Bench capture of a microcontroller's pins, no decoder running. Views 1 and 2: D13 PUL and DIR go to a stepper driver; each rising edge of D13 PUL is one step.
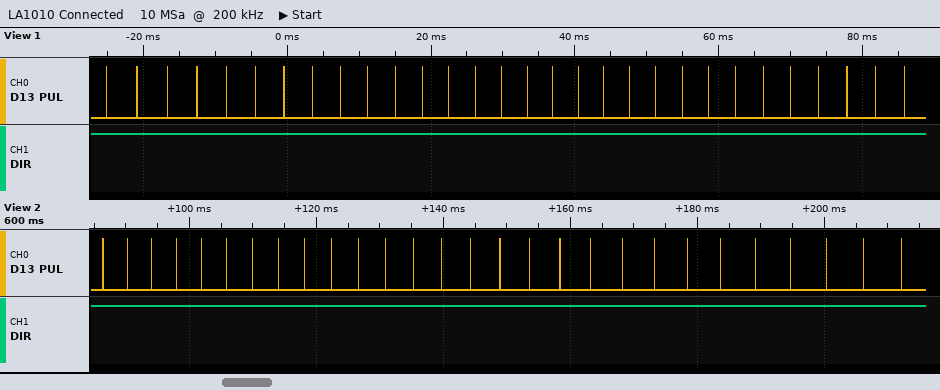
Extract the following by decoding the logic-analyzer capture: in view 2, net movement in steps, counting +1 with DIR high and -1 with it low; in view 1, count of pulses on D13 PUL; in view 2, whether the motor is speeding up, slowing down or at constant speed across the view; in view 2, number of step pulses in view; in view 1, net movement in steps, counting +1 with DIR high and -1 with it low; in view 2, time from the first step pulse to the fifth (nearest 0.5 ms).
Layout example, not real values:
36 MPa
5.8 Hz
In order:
+28
30
slowing down
28
+30
15.5 ms
